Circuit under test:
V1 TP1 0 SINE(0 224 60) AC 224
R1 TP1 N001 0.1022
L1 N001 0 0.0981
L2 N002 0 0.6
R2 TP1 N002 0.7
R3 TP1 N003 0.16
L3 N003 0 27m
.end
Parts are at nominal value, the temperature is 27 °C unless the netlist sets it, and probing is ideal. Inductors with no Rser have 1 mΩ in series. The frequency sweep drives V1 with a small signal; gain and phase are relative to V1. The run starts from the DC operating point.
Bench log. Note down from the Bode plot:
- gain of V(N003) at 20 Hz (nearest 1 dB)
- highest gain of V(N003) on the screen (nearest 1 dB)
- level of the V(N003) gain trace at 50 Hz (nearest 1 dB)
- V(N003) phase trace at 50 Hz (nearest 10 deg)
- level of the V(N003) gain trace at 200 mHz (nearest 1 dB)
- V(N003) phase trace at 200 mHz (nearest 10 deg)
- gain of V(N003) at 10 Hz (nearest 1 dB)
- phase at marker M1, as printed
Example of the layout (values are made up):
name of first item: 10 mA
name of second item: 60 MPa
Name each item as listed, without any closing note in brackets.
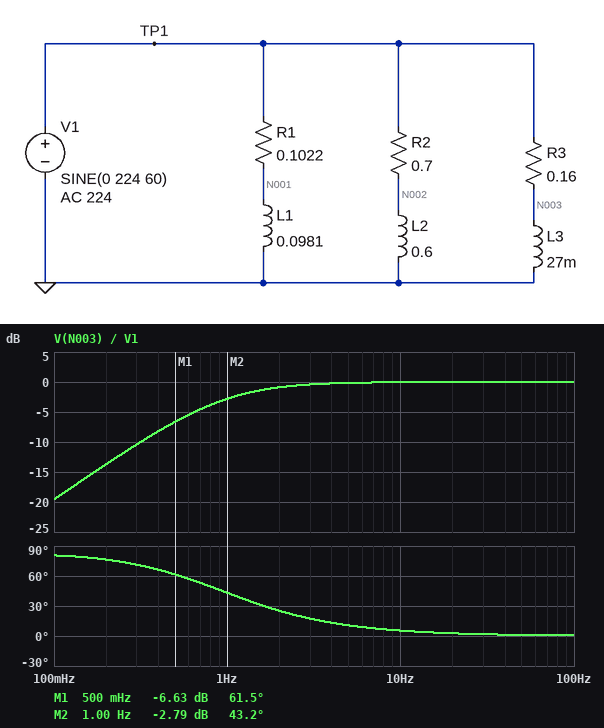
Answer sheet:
gain of V(N003) at 20 Hz: 0 dB
highest gain of V(N003) on the screen: 0 dB
level of the V(N003) gain trace at 50 Hz: 0 dB
V(N003) phase trace at 50 Hz: 0 deg
level of the V(N003) gain trace at 200 mHz: -14 dB
V(N003) phase trace at 200 mHz: 80 deg
gain of V(N003) at 10 Hz: 0 dB
phase at marker M1, as printed: 61.5 deg
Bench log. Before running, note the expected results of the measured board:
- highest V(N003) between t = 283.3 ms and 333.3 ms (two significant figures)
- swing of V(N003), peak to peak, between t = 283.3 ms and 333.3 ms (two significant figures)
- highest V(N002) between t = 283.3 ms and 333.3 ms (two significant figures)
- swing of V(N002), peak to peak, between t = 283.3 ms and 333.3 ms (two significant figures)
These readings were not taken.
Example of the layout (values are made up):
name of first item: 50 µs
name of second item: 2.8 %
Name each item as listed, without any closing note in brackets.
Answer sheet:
highest V(N003) between t = 283.3 ms and 333.3 ms: 220 V
swing of V(N003), peak to peak, between t = 283.3 ms and 333.3 ms: 450 V
highest V(N002) between t = 283.3 ms and 333.3 ms: 220 V
swing of V(N002), peak to peak, between t = 283.3 ms and 333.3 ms: 450 V
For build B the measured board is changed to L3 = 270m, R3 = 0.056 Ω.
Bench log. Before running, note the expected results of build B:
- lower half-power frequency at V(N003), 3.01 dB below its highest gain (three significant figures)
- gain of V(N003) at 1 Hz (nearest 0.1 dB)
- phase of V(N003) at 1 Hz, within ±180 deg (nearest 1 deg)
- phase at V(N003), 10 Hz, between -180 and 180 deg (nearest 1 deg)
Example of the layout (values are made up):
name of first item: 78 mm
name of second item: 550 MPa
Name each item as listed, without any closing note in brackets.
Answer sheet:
lower half-power frequency at V(N003), 3.01 dB below its highest gain: 33.6 mHz
gain of V(N003) at 1 Hz: 0 dB
phase of V(N003) at 1 Hz, within ±180 deg: 2 deg
phase at V(N003), 10 Hz, between -180 and 180 deg: 0 deg
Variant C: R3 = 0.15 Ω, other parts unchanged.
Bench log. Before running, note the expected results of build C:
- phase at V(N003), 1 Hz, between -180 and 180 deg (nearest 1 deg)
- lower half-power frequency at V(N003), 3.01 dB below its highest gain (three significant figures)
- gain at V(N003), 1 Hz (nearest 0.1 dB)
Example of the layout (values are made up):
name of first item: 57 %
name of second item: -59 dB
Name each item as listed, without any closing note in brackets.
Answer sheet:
phase at V(N003), 1 Hz, between -180 and 180 deg: 41 deg
lower half-power frequency at V(N003), 3.01 dB below its highest gain: 890 mHz
gain at V(N003), 1 Hz: -2.5 dB
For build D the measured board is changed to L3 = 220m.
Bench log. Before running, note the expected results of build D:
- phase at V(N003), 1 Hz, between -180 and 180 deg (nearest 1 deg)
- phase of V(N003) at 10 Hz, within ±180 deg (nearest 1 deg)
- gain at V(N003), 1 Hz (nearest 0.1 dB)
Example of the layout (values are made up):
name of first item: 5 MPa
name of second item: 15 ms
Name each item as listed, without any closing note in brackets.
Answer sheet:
phase at V(N003), 1 Hz, between -180 and 180 deg: 7 deg
phase of V(N003) at 10 Hz, within ±180 deg: 1 deg
gain at V(N003), 1 Hz: -0.1 dB
